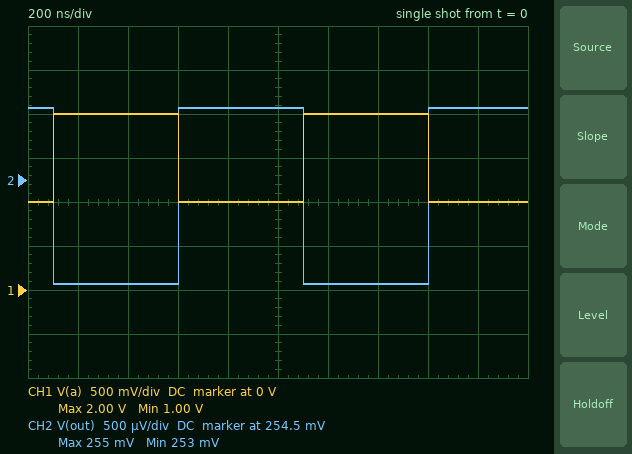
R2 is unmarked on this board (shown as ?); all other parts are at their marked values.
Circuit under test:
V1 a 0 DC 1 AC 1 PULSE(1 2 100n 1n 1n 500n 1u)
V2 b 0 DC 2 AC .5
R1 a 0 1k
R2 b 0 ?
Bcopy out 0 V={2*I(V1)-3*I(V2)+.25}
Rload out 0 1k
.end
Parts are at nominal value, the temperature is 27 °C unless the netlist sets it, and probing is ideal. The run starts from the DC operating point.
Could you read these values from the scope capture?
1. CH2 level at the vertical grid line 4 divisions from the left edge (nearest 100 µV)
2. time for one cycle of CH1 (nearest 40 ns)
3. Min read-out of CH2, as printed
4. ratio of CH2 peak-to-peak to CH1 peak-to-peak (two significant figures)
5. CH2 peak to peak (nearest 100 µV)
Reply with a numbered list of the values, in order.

1. 255.3 mV
2. 1.00 µs
3. 253 mV
4. 0.0020
5. 2.0 mV
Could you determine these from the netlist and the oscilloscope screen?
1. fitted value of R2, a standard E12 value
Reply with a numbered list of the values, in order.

1. 820 Ω
